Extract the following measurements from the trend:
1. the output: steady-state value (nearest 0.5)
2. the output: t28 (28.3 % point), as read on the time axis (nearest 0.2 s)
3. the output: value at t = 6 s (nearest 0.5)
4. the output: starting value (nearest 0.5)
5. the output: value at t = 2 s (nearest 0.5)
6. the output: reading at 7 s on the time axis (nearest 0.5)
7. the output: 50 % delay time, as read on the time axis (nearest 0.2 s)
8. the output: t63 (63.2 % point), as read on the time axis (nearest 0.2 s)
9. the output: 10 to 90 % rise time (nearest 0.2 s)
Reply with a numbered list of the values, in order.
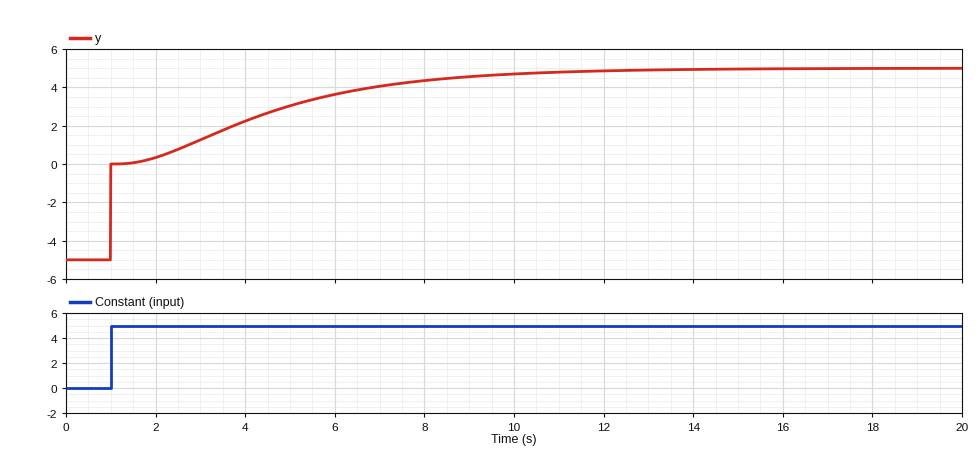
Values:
1. 5.0
2. 1.0 s
3. 3.5
4. -5.0
5. 0.5
6. 4.0
7. 1.0 s
8. 3.0 s
9. 5.8 s
